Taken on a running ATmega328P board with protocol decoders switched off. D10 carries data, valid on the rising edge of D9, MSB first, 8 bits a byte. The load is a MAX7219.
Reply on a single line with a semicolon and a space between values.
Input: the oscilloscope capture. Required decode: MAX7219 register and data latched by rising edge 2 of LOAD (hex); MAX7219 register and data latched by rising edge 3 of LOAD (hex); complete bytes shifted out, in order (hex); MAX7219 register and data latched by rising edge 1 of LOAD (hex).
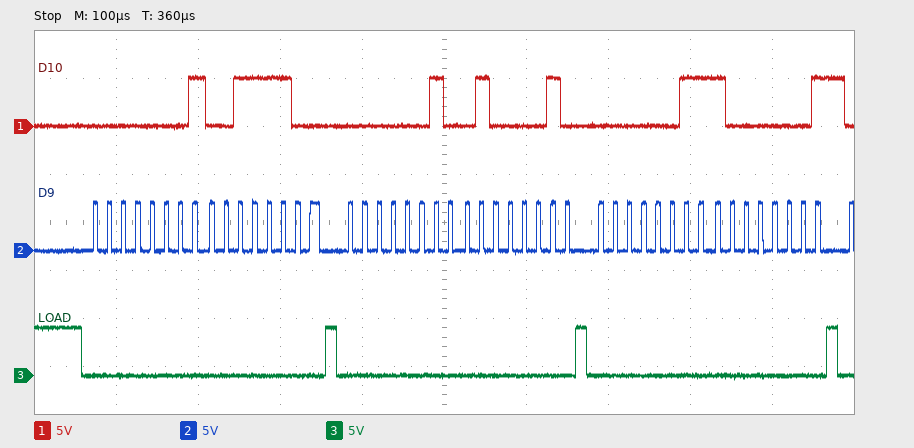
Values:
register 0x2, data 0x42; register 0x3, data 0x81; 01 3C 02 42 03 81; register 0x1, data 0x3C
